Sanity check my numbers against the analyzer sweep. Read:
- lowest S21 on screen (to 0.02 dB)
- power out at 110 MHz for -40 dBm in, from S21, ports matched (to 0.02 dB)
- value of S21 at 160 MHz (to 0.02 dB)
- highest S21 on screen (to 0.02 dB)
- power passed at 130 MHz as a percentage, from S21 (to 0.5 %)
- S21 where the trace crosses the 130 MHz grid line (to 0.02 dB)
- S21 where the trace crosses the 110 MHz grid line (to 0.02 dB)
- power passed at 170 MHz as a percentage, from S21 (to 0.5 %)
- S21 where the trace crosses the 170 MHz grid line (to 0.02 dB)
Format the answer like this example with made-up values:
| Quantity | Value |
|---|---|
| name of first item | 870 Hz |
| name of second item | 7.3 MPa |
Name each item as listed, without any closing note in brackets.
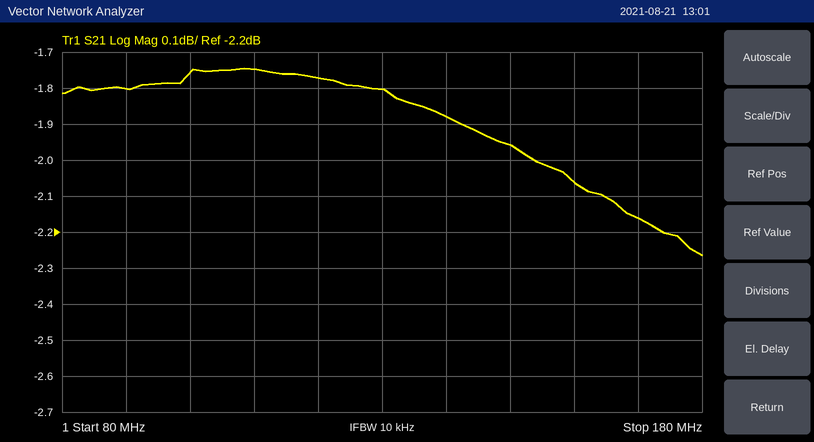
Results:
| Quantity | Value |
|---|---|
| lowest S21 on screen | -2.26 dB |
| power out at 110 MHz for -40 dBm in, from S21, ports matched | -41.74 dBm |
| value of S21 at 160 MHz | -2.06 dB |
| highest S21 on screen | -1.74 dB |
| power passed at 130 MHz as a percentage, from S21 | 66.0 % |
| S21 where the trace crosses the 130 MHz grid line | -1.80 dB |
| S21 where the trace crosses the 110 MHz grid line | -1.74 dB |
| power passed at 170 MHz as a percentage, from S21 | 61.0 % |
| S21 where the trace crosses the 170 MHz grid line | -2.16 dB |
